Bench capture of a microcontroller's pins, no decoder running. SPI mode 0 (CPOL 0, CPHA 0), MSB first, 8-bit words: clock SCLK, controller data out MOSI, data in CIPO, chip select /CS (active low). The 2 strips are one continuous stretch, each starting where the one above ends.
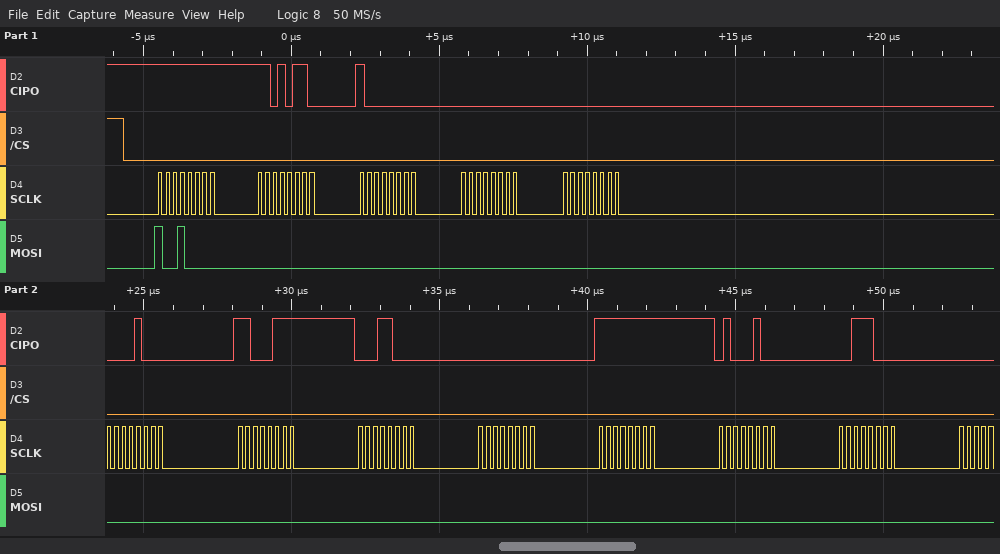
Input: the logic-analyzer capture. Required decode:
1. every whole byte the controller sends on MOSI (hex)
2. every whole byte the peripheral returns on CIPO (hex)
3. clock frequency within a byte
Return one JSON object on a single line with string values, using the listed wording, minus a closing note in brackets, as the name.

{"every whole byte the controller sends on MOSI": "0x90 0x00 0x00 0x00 0x00 0x00 0x00 0x00 0x00 0x00 0x00 0x00", "every whole byte the peripheral returns on CIPO": "0xFF 0xD6 0x80 0x00 0x00 0x08 0xC7 0x18 0x00 0xFF 0x44 0x38", "clock frequency within a byte": "4 MHz"}
